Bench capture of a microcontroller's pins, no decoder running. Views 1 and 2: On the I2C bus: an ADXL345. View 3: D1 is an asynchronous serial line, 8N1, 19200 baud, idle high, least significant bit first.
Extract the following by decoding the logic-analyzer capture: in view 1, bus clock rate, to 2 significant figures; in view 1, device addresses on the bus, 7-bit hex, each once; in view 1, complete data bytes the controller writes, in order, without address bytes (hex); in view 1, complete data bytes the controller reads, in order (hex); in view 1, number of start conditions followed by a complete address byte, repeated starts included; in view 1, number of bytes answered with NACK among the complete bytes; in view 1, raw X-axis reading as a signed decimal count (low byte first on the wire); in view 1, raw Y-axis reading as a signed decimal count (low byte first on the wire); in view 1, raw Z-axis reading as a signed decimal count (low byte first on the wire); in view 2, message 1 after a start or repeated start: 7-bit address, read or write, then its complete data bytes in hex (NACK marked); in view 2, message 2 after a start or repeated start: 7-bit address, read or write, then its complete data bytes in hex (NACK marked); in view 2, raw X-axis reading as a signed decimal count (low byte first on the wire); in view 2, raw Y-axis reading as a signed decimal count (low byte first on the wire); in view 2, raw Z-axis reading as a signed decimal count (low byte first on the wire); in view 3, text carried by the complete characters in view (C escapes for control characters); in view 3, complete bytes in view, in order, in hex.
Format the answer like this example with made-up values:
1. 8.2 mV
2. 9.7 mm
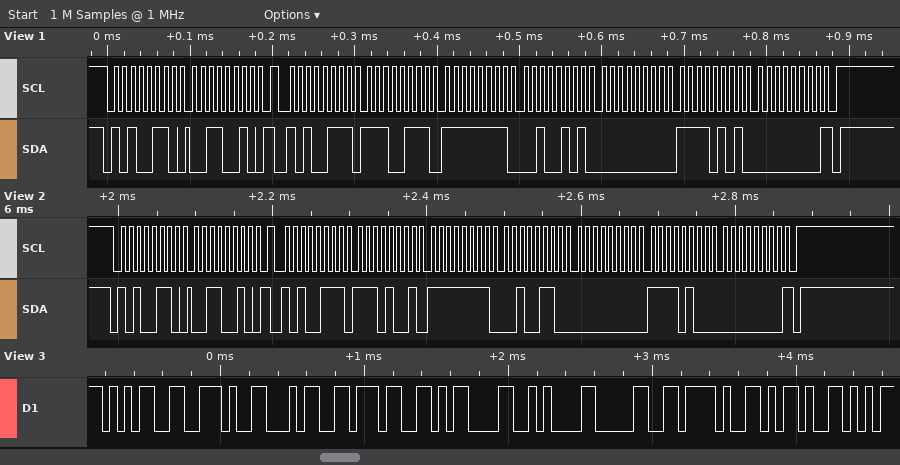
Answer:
1. 100 kHz
2. 0x53
3. 32
4. E7 FF 25 00 F5 00
5. 2
6. 1
7. -25
8. 37
9. 245
10. 0x53 write: 32
11. 0x53 read: E9 FF 26 00 F4 00 NACK
12. -23
13. 38
14. 244
15. "5.47\r\n0/-"
16. 0x35 0x2E 0x34 0x37 0x0D 0x0A 0x30 0x2F 0x2D
